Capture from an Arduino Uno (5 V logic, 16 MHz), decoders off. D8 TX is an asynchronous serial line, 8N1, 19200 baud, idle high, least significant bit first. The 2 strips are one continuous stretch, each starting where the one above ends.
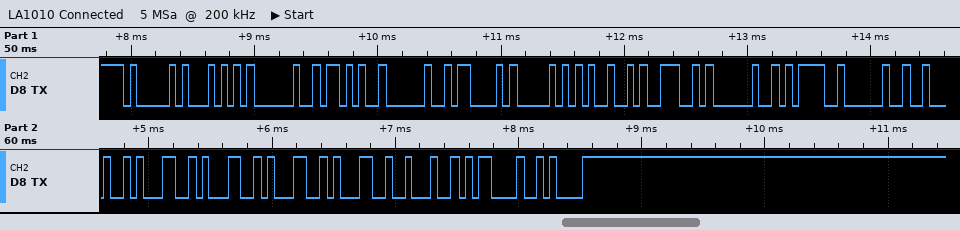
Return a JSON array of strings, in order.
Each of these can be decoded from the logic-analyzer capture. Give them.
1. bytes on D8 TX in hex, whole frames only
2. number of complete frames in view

["0x41 0x54 0x20 0x2B 0x20 0x43 0x50 0x49 0x4E 0x20 0x3D 0x20 0x22 0x31 0x31 0x31 0x31 0x22 0x0D 0x0A", "20"]
